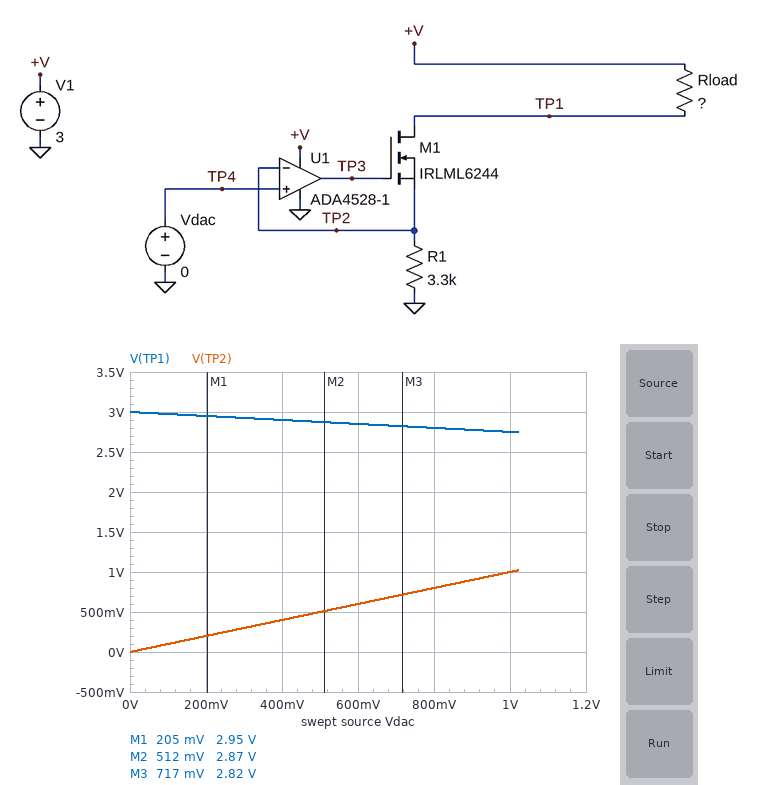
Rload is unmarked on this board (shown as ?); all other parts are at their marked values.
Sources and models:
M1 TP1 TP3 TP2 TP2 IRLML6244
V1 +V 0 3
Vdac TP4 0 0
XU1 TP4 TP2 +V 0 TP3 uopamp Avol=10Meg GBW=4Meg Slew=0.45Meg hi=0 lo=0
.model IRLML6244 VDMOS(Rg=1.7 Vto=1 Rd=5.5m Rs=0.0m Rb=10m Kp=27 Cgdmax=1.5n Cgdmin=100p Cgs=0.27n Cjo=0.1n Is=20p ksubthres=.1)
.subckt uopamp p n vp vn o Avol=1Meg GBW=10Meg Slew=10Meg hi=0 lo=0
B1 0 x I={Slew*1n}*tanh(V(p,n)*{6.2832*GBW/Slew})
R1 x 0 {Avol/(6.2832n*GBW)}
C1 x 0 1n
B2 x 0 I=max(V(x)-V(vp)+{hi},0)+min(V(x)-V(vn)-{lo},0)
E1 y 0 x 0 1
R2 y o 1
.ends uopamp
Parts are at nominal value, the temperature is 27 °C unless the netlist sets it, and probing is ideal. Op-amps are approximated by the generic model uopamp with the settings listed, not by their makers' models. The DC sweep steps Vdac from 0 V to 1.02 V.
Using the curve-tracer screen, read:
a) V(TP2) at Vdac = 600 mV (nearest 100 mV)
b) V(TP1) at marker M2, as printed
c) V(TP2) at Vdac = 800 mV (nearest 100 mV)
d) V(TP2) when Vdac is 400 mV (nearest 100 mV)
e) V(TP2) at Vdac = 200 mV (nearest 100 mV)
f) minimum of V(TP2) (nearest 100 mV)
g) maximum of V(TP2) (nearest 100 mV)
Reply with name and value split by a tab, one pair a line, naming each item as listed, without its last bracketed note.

V(TP2) at Vdac = 600 mV	600 mV
V(TP1) at marker M2, as printed	2.87 V
V(TP2) at Vdac = 800 mV	800 mV
V(TP2) when Vdac is 400 mV	400 mV
V(TP2) at Vdac = 200 mV	200 mV
minimum of V(TP2)	0 V
maximum of V(TP2)	1.0 V
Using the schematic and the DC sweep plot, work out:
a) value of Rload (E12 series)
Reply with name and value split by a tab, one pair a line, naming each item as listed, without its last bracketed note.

value of Rload	820 Ω
